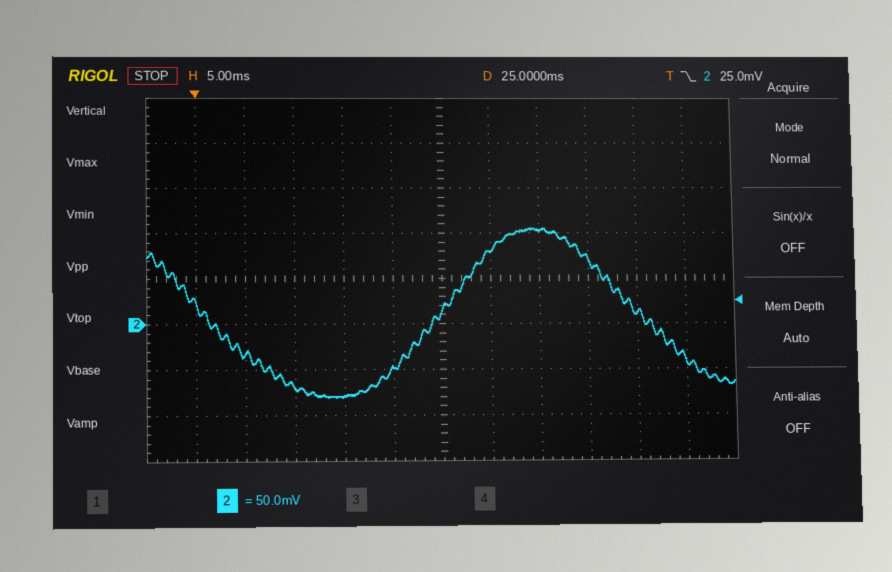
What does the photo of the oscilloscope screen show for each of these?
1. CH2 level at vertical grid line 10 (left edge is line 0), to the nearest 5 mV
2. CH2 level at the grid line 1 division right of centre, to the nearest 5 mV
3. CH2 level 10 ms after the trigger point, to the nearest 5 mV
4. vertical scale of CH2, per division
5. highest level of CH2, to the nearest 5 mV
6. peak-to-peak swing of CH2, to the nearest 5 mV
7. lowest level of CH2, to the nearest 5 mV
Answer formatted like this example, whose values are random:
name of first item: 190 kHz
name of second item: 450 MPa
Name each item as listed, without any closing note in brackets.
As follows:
CH2 level at vertical grid line 10 (left edge is line 0), to the nearest 5 mV: 15 mV
CH2 level at the grid line 1 division right of centre, to the nearest 5 mV: 80 mV
CH2 level 10 ms after the trigger point, to the nearest 5 mV: -70 mV
vertical scale of CH2, per division: 50 mV
highest level of CH2, to the nearest 5 mV: 105 mV
peak-to-peak swing of CH2, to the nearest 5 mV: 185 mV
lowest level of CH2, to the nearest 5 mV: -80 mV
